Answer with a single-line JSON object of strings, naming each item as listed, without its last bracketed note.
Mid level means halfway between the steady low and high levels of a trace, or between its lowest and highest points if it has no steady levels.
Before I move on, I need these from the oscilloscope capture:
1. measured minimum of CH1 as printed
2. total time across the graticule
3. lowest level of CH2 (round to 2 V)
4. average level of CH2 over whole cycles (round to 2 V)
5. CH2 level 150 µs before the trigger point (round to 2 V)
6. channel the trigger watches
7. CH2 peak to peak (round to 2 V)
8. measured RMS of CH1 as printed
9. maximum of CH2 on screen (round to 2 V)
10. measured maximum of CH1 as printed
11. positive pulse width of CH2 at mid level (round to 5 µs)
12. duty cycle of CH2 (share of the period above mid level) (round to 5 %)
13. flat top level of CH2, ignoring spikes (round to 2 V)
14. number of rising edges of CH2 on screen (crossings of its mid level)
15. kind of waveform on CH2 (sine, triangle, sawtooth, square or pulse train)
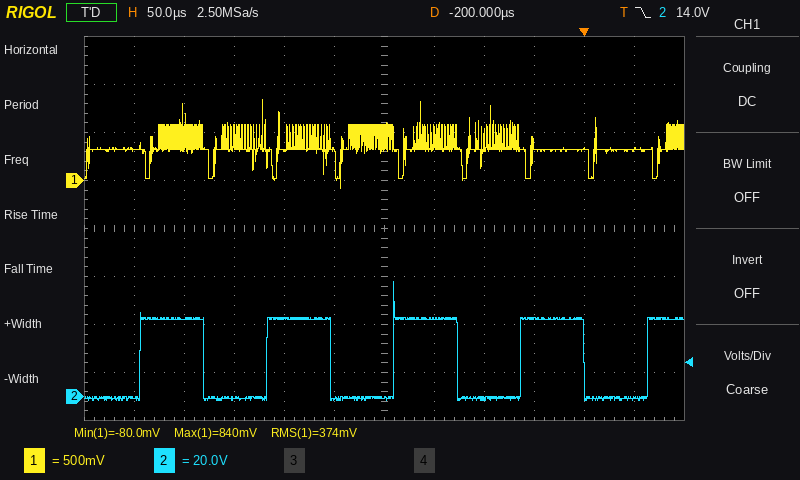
{"measured minimum of CH1 as printed": "-80.0 mV", "total time across the graticule": "600 µs", "lowest level of CH2": "-2 V", "average level of CH2 over whole cycles": "16 V", "CH2 level 150 µs before the trigger point": "32 V", "channel the trigger watches": "CH2", "CH2 peak to peak": "50 V", "measured RMS of CH1 as printed": "374 mV", "maximum of CH2 on screen": "48 V", "measured maximum of CH1 as printed": "840 mV", "positive pulse width of CH2 at mid level": "65 µs", "duty cycle of CH2 (share of the period above mid level)": "50 %", "flat top level of CH2, ignoring spikes": "32 V", "number of rising edges of CH2 on screen": "5", "kind of waveform on CH2": "square"}
